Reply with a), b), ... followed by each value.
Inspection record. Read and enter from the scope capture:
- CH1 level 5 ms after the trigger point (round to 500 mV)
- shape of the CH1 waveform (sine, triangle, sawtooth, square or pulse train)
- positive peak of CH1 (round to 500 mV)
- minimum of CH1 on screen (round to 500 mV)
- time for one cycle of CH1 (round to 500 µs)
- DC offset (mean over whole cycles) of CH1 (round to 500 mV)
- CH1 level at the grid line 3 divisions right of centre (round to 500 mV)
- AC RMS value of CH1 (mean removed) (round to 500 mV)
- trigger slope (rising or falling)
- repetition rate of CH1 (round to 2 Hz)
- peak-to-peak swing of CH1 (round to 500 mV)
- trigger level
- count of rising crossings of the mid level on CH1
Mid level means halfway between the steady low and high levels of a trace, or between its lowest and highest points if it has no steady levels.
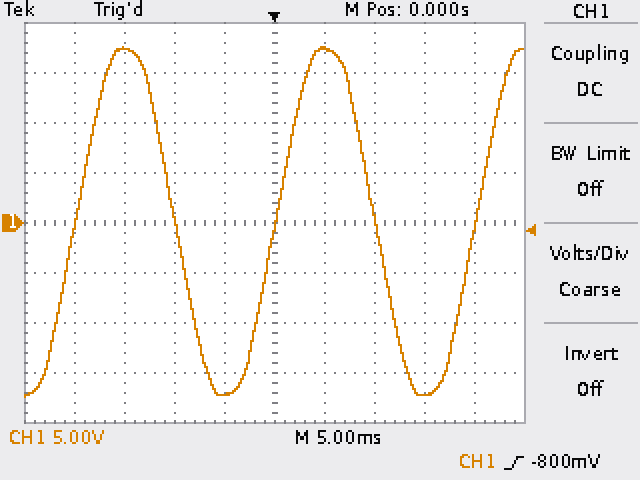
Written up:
a) 17.5 V
b) sine
c) 17.5 V
d) -17.5 V
e) 20.0 ms
f) 0.0 V
g) -17.0 V
h) 12.5 V
i) rising
j) 50 Hz
k) 35.0 V
l) -800 mV
m) 3
